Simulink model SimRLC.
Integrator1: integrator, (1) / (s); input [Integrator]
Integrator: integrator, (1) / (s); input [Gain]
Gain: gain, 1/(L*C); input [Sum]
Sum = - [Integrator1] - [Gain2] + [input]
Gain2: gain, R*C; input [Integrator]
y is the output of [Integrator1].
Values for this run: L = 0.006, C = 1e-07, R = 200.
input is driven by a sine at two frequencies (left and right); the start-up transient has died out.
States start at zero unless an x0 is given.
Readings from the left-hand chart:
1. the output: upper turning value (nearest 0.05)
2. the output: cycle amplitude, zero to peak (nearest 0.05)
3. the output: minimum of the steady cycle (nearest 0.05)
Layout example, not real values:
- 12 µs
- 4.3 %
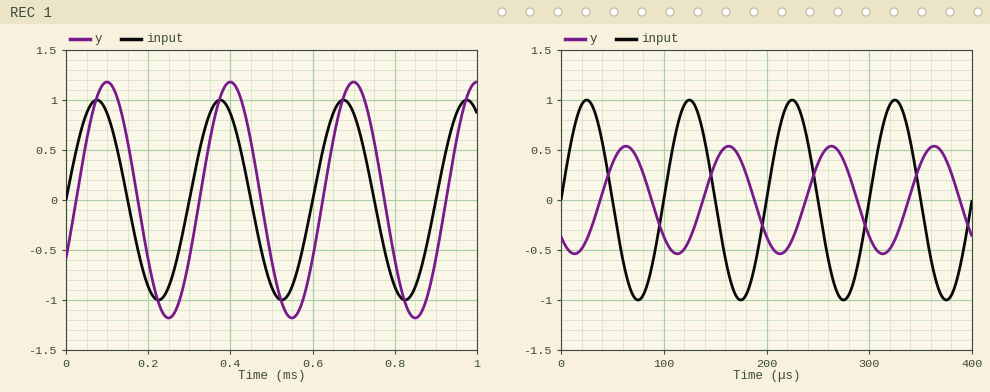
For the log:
- 1.20
- 1.20
- -1.20
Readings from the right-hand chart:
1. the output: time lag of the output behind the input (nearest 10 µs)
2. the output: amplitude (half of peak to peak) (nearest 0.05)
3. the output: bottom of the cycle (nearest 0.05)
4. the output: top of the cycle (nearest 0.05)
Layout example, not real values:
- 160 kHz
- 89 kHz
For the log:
- 40 µs
- 0.55
- -0.55
- 0.55
